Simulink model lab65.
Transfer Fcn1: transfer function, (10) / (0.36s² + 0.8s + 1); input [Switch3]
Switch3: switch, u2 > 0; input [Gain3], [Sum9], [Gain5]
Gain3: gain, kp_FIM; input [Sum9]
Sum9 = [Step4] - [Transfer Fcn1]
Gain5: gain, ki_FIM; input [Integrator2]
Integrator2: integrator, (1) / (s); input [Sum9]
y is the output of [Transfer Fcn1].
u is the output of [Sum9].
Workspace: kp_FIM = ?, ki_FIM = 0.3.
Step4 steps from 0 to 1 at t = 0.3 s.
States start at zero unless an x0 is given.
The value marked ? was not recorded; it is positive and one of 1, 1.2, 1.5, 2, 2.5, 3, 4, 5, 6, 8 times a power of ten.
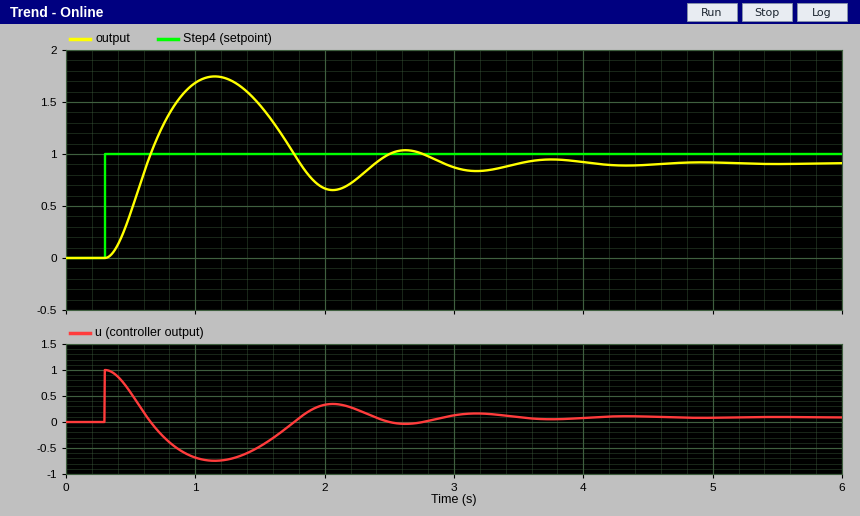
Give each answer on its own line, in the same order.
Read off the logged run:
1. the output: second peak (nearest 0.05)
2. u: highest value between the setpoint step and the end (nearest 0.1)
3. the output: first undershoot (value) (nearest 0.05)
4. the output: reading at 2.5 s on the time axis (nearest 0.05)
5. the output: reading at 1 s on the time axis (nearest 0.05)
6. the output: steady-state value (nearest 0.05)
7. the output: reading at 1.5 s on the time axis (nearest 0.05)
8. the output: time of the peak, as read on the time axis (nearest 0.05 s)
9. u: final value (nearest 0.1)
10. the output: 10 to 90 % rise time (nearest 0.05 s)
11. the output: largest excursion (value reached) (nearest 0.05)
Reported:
1.05
1.0
0.65
1.00
1.70
0.90
1.45
1.15 s
0.1
0.20 s
1.75
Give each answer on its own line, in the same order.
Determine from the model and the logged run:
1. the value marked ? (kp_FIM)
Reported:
1
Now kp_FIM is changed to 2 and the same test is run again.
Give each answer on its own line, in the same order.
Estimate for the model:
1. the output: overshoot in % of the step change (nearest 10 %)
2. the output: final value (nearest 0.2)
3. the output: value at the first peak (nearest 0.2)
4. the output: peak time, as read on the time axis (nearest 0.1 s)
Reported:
140 %
1.0
2.2
1.0 s
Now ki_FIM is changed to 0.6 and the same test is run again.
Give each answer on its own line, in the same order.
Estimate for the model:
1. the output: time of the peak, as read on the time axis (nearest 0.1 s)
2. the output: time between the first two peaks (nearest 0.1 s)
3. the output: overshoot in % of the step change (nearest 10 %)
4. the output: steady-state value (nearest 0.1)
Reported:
1.2 s
1.4 s
100 %
0.9
